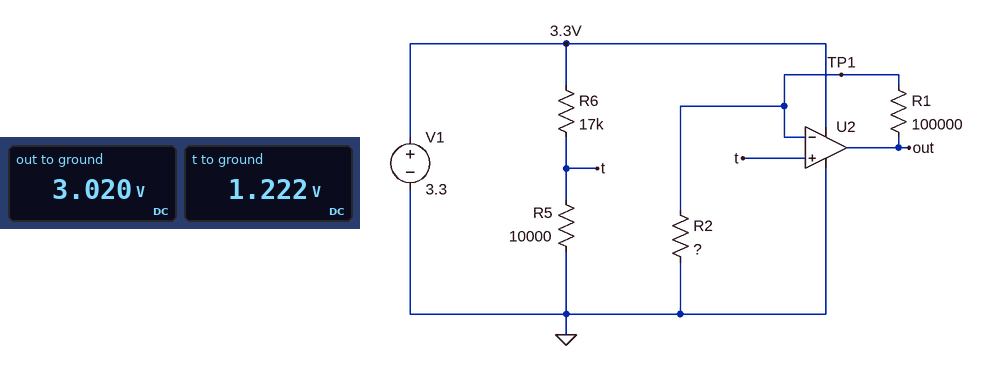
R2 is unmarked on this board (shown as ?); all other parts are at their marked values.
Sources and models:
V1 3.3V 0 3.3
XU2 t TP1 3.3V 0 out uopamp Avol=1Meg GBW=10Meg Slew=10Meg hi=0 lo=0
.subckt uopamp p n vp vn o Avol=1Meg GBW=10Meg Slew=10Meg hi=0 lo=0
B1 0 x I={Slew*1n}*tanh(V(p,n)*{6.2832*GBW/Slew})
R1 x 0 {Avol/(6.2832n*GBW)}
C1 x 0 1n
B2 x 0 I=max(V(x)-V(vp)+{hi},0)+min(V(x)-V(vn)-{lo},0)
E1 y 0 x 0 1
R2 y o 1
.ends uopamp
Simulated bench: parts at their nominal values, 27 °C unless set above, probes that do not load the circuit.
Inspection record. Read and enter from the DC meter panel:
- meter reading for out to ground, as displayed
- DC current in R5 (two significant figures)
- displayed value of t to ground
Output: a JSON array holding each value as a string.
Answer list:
["3.020 V", "120 µA", "1.222 V"]
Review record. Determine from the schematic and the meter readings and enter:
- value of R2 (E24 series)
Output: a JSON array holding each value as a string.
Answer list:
["68 kΩ"]
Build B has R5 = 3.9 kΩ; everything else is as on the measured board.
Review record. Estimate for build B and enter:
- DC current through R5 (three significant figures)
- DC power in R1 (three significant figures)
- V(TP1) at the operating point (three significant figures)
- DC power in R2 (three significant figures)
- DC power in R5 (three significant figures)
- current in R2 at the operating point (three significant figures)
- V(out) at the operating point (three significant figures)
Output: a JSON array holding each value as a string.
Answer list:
["158 µA", "8.20 µW", "616 mV", "5.58 µW", "97.2 µW", "9.06 µA", "1.52 V"]
